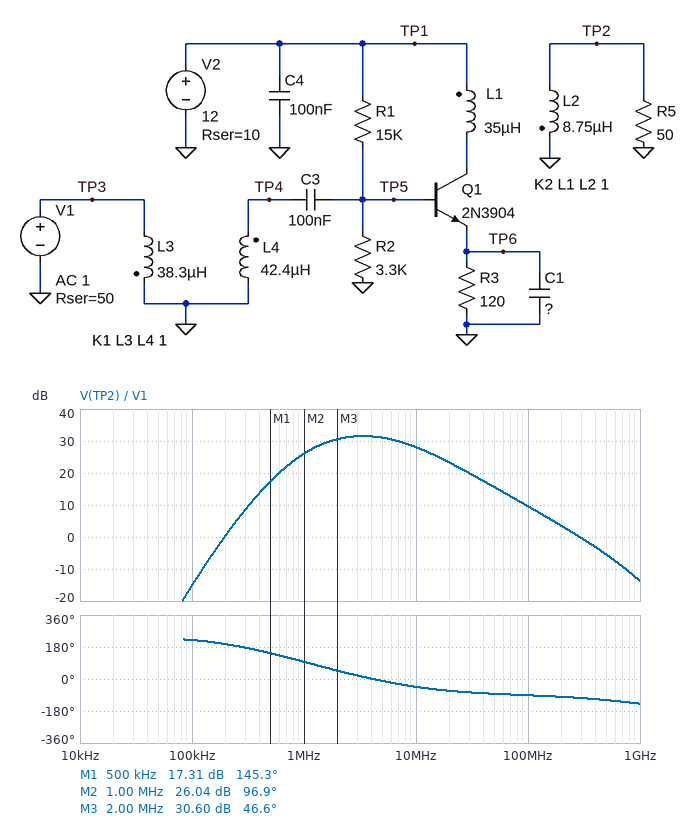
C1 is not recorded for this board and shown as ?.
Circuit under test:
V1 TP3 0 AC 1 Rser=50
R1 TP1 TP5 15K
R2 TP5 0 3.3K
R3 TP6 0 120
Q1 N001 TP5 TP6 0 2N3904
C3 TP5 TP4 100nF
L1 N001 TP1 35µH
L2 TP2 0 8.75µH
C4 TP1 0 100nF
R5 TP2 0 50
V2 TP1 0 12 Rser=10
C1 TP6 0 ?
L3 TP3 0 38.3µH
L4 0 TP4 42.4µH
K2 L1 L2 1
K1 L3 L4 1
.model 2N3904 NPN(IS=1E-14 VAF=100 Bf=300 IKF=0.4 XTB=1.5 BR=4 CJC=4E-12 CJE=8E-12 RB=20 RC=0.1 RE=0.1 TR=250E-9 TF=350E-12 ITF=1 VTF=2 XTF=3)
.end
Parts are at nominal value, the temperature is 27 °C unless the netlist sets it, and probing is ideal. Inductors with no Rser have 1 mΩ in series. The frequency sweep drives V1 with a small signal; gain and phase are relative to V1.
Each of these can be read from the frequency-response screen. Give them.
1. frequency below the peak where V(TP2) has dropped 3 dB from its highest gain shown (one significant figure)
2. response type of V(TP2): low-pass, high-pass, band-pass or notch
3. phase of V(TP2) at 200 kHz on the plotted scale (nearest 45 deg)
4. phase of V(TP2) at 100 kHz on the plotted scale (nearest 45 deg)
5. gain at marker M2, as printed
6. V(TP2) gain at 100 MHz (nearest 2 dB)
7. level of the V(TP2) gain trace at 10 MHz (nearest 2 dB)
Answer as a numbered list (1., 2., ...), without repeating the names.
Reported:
1. 1 MHz
2. band-pass
3. 180 deg
4. 225 deg
5. 26.04 dB
6. 10 dB
7. 28 dB
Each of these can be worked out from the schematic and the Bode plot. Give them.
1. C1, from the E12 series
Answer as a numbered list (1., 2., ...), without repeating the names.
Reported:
1. 56 nF
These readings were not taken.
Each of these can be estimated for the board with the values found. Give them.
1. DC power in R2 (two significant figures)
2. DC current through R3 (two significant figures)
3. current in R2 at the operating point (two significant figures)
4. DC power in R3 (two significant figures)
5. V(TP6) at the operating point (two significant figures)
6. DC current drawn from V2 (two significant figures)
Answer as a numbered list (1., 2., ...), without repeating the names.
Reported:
1. 1.3 mW
2. 11 mA
3. 620 µA
4. 15 mW
5. 1.3 V
6. 12 mA
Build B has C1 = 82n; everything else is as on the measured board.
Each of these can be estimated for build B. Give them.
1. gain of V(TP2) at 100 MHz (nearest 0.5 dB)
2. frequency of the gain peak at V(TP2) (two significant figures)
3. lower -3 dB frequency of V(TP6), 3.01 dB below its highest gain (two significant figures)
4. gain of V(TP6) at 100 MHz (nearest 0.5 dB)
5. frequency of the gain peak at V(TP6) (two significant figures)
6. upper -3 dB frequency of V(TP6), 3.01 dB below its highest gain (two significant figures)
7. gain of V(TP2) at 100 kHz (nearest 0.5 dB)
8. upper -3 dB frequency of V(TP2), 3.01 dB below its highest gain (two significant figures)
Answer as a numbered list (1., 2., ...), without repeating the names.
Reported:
1. 9.5 dB
2. 3.1 MHz
3. 140 kHz
4. -64.0 dB
5. 400 kHz
6. 1.2 MHz
7. -12.0 dB
8. 9.2 MHz
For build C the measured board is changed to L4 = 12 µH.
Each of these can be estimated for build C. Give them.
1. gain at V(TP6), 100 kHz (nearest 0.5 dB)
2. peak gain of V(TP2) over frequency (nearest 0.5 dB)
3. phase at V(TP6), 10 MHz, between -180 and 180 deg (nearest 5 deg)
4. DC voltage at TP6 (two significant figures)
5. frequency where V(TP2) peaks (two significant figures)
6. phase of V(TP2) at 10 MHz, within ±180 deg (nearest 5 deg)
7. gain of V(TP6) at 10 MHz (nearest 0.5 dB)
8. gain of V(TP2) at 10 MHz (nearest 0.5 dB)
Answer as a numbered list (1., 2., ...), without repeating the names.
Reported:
1. -12.5 dB
2. 26.5 dB
3. 65 deg
4. 1.3 V
5. 4.8 MHz
6. -20 deg
7. -25.5 dB
8. 25.5 dB
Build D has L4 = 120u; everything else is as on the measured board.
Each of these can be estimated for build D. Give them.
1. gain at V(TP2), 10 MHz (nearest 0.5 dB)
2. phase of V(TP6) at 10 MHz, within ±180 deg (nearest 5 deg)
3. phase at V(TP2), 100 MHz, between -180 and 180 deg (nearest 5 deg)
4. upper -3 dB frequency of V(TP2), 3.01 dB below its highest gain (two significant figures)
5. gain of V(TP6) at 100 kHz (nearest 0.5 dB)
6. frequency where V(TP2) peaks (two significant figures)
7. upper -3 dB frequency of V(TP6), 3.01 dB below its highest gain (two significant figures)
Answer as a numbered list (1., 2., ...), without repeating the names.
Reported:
1. 26.5 dB
2. 25 deg
3. -95 deg
4. 4.9 MHz
5. -2.5 dB
6. 2.3 MHz
7. 1.7 MHz
